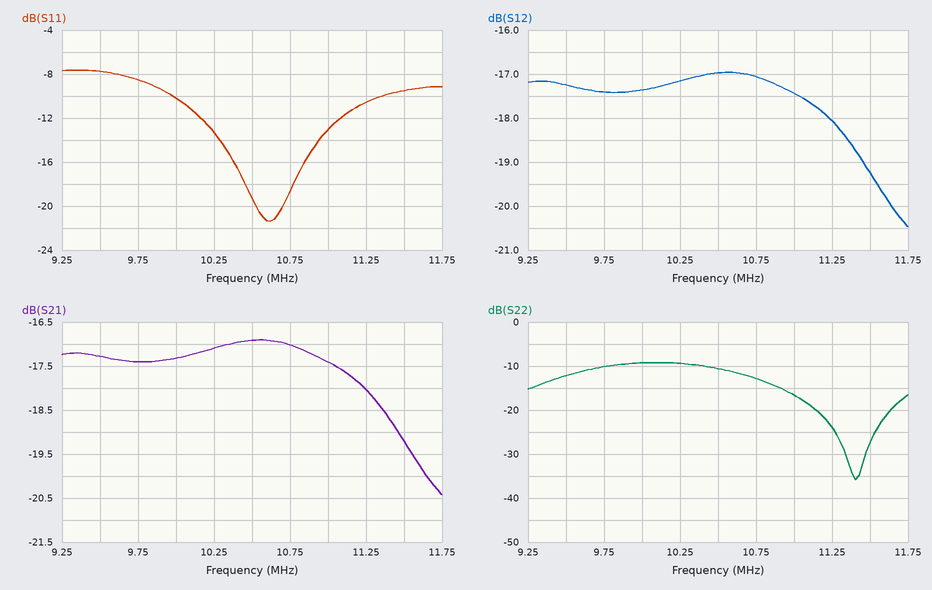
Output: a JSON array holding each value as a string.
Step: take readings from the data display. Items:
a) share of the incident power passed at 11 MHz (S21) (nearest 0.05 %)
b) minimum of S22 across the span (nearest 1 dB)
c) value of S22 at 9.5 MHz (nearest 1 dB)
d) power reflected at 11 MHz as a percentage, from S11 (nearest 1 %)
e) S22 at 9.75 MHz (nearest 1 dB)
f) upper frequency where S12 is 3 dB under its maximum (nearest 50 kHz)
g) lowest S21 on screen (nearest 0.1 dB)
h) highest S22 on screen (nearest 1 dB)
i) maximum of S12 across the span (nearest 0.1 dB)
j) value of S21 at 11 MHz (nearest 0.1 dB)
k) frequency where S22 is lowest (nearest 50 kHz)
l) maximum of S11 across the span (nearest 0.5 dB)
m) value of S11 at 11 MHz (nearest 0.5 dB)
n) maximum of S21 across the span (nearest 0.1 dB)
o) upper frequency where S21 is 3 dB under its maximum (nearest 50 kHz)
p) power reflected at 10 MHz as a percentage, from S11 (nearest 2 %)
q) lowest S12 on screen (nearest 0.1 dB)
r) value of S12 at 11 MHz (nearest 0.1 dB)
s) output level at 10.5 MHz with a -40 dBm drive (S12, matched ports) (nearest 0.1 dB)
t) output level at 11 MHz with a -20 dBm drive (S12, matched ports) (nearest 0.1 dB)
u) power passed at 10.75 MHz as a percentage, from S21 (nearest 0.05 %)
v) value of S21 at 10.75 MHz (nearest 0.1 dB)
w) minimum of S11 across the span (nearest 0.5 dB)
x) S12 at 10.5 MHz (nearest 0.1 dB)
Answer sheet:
["1.80 %", "-36 dB", "-12 dB", "5 %", "-10 dB", "11.65 MHz", "-20.4 dB", "-9 dB", "-17.0 dB", "-17.4 dB", "11.40 MHz", "-7.5 dB", "-13.0 dB", "-16.9 dB", "11.65 MHz", "10 %", "-20.5 dB", "-17.4 dB", "-57.0 dBm", "-37.4 dBm", "2.00 %", "-17.0 dB", "-21.5 dB", "-17.0 dB"]
